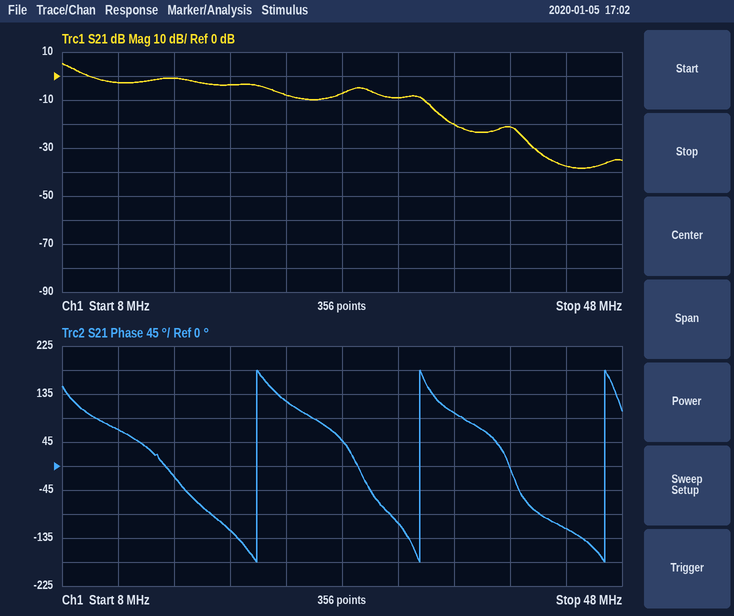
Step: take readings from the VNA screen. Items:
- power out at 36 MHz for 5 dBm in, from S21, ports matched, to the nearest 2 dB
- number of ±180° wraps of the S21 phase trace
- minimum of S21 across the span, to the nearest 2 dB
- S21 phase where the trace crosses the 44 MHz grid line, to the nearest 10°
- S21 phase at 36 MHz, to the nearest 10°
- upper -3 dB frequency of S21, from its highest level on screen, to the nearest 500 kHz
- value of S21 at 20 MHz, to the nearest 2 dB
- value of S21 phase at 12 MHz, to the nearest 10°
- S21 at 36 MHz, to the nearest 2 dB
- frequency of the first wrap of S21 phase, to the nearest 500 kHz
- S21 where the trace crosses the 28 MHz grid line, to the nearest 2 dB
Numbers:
-16 dBm
3
-38 dB
-120°
100°
9.0 MHz
-4 dB
70°
-20 dB
22.0 MHz
-8 dB
